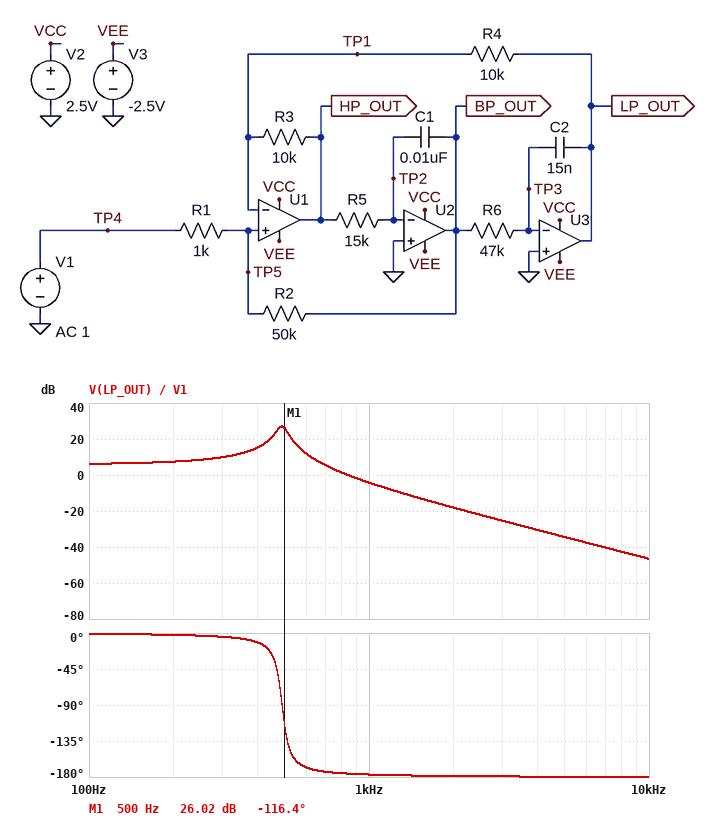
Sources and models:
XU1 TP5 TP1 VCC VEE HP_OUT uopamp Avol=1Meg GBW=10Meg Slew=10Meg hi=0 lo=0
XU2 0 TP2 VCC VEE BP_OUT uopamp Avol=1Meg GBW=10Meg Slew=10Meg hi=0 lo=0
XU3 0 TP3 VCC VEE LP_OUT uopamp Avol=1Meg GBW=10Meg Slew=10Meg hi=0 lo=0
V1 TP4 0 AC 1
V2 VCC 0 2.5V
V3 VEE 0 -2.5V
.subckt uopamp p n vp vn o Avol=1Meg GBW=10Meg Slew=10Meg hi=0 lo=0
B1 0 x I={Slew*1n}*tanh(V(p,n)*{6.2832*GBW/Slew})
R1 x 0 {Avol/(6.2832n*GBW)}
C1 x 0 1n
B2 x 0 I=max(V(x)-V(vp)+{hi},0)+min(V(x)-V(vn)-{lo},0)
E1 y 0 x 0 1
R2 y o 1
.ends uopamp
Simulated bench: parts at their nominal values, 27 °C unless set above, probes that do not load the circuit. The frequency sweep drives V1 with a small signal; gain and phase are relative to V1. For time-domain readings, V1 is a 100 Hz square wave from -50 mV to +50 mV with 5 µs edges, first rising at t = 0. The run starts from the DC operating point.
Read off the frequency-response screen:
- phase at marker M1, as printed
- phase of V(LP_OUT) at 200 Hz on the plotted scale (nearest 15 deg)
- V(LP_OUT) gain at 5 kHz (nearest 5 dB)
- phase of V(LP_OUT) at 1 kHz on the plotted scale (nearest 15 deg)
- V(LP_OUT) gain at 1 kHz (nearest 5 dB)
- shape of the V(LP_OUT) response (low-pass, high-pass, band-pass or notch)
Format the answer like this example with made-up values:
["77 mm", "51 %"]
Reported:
["-116.4 deg", "0 deg", "-35 dB", "-180 deg", "-5 dB", "low-pass"]
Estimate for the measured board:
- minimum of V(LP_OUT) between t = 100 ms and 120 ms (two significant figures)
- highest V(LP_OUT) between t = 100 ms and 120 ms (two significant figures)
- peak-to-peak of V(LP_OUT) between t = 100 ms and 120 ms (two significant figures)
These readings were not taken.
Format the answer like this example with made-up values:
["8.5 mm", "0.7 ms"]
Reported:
["-410 mV", "410 mV", "820 mV"]
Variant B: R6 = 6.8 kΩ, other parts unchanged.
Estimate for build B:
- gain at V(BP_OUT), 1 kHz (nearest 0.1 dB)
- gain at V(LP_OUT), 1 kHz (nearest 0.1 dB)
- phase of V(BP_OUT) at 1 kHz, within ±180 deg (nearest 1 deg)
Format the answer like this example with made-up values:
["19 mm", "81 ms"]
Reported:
["10.0 dB", "13.9 dB", "-94 deg"]
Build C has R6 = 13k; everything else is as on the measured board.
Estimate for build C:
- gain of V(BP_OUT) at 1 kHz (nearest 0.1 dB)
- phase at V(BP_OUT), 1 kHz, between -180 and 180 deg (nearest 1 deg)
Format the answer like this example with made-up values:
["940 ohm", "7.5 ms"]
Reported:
["23.4 dB", "107 deg"]
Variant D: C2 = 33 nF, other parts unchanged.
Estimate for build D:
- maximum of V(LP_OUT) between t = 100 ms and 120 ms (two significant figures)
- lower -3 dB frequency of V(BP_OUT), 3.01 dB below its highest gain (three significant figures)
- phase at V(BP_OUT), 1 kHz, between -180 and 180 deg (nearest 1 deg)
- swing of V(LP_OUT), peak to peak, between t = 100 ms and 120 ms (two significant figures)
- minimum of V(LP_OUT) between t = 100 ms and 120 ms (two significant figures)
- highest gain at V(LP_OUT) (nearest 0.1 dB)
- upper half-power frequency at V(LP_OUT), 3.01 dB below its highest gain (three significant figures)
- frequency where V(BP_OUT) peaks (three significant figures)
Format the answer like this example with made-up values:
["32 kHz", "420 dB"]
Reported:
["310 mV", "310 Hz", "93 deg", "610 mV", "-310 mV", "23.9 dB", "349 Hz", "330 Hz"]
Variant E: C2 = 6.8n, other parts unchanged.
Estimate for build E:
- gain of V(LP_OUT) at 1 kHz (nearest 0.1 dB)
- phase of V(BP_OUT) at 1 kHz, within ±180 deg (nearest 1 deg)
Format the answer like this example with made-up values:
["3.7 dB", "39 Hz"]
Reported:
["6.8 dB", "95 deg"]
